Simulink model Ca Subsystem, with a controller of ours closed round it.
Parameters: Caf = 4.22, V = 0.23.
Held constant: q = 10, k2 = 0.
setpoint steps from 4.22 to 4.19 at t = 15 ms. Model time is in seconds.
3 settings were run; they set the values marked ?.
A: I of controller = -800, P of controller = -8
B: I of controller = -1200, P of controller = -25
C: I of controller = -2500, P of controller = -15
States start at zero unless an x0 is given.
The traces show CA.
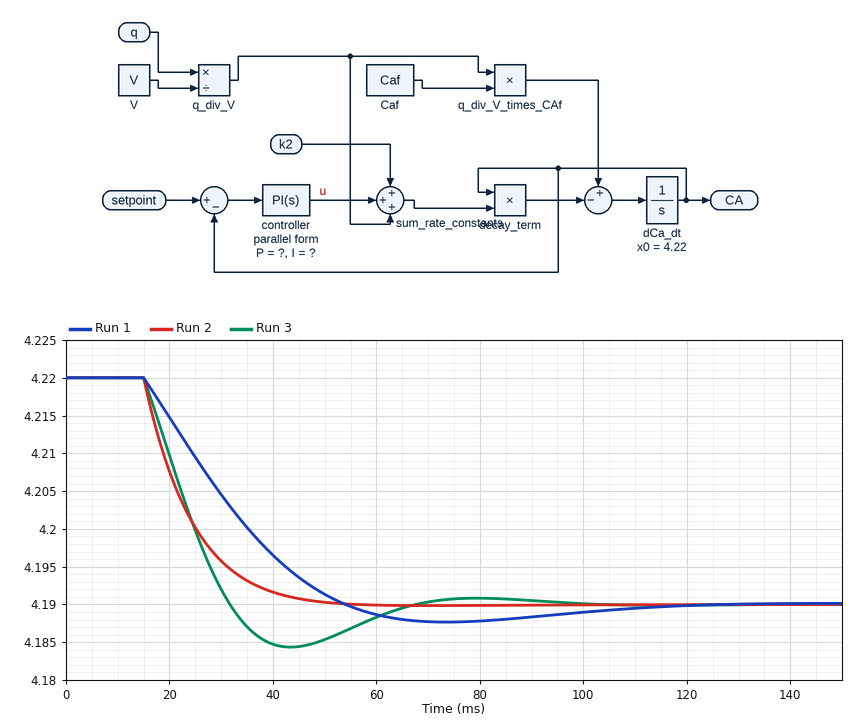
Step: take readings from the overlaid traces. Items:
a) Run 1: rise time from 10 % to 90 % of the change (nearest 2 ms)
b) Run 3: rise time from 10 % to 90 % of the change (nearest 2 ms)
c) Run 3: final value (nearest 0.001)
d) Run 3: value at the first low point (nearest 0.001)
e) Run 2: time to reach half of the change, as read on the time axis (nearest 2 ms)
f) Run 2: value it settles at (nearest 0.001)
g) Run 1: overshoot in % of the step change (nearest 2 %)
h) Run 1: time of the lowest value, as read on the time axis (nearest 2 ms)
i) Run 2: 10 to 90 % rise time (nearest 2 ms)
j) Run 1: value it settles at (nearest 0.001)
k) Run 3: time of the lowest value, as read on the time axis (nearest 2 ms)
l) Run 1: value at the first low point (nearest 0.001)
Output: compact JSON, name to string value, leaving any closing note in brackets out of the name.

{"Run 1: rise time from 10 % to 90 % of the change": "28 ms", "Run 3: rise time from 10 % to 90 % of the change": "12 ms", "Run 3: final value": "4.190", "Run 3: value at the first low point": "4.184", "Run 2: time to reach half of the change, as read on the time axis": "22 ms", "Run 2: value it settles at": "4.190", "Run 1: overshoot in % of the step change": "8 %", "Run 1: time of the lowest value, as read on the time axis": "74 ms", "Run 2: 10 to 90 % rise time": "20 ms", "Run 1: value it settles at": "4.190", "Run 3: time of the lowest value, as read on the time axis": "44 ms", "Run 1: value at the first low point": "4.188"}
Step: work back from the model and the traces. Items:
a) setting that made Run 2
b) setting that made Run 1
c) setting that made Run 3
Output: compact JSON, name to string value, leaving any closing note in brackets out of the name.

{"setting that made Run 2": "B", "setting that made Run 1": "A", "setting that made Run 3": "C"}
